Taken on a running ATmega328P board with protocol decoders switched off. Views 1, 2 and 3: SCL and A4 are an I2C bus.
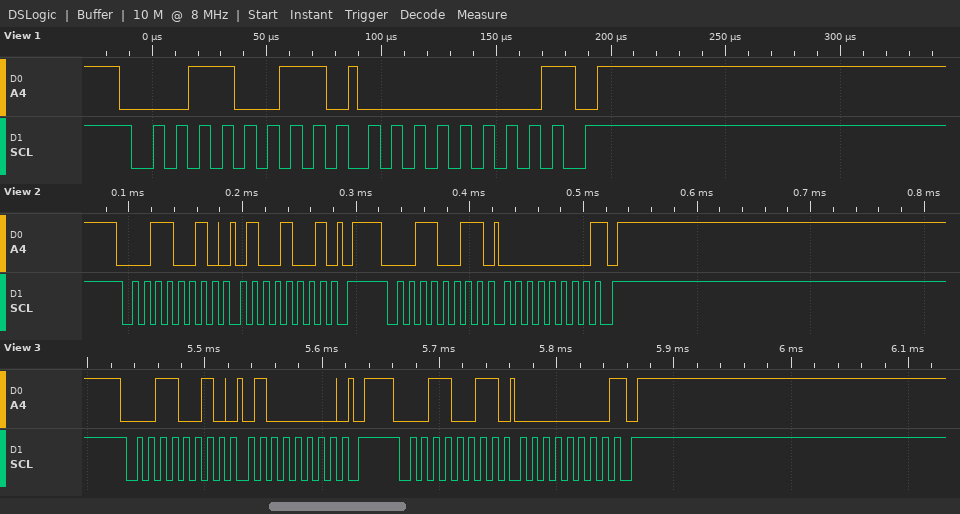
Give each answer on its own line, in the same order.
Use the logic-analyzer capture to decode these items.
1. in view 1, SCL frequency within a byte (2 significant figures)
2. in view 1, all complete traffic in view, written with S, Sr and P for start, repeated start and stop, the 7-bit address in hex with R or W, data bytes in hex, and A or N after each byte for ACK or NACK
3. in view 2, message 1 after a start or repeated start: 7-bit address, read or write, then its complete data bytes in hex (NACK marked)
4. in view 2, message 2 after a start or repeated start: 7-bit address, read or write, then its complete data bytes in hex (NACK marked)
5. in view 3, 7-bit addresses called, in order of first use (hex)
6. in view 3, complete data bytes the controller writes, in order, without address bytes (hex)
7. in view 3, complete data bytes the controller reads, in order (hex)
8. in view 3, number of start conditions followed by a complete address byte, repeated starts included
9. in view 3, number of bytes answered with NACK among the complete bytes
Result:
100 kHz
S 19R A 00 N P
0x19 write: 49
0x19 read: 00 NACK
0x19
40
00
2
1
